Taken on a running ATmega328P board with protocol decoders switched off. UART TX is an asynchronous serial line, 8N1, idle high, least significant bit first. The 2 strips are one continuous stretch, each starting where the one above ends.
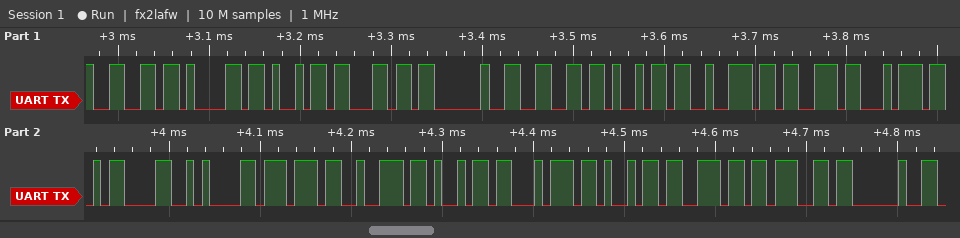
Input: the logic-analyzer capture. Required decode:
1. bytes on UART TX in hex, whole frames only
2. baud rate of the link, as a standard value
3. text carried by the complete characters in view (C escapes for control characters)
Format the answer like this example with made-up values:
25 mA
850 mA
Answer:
0x66 0x61 0x69 0x6C 0x20 0x66 0x69 0x72 0x73 0x74 0x0D 0x0A 0x77 0x72 0x69 0x74 0x69 0x6E 0x67 0x20
115200 baud
"fail first\r\nwriting "
